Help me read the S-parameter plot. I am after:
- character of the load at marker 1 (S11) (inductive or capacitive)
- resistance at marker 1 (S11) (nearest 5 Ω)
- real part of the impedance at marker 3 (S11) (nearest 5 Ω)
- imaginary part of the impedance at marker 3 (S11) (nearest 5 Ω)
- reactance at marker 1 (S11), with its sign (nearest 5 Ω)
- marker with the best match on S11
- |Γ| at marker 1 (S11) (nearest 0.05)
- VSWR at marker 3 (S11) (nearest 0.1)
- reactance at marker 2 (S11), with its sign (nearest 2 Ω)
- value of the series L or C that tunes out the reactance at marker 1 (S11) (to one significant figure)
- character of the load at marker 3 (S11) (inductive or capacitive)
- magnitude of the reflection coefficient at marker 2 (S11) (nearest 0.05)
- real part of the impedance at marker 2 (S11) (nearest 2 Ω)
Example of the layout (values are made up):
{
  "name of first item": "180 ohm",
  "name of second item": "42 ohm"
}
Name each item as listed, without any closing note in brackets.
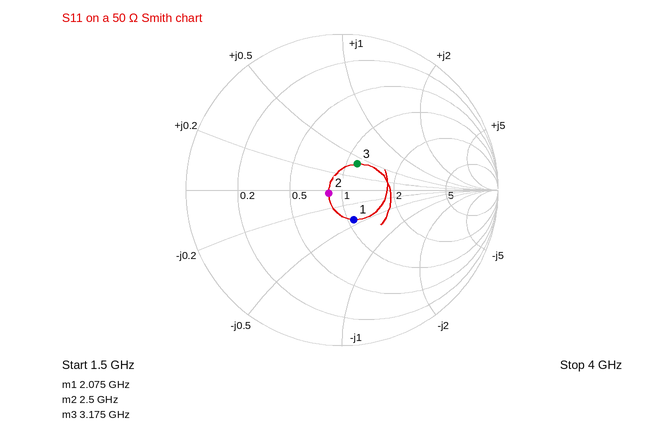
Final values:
{
  "character of the load at marker 1 (S11)": "capacitive",
  "resistance at marker 1 (S11)": "55 Ω",
  "real part of the impedance at marker 3 (S11)": "55 Ω",
  "imaginary part of the impedance at marker 3 (S11)": "+20 Ω",
  "reactance at marker 1 (S11), with its sign": "-20 Ω",
  "marker with the best match on S11": "marker 2",
  "|Γ| at marker 1 (S11)": "0.20",
  "VSWR at marker 3 (S11)": "1.5",
  "reactance at marker 2 (S11), with its sign": "-2 Ω",
  "value of the series L or C that tunes out the reactance at marker 1 (S11)": "2 nH",
  "character of the load at marker 3 (S11)": "inductive",
  "magnitude of the reflection coefficient at marker 2 (S11)": "0.10",
  "real part of the impedance at marker 2 (S11)": "42 Ω"
}
